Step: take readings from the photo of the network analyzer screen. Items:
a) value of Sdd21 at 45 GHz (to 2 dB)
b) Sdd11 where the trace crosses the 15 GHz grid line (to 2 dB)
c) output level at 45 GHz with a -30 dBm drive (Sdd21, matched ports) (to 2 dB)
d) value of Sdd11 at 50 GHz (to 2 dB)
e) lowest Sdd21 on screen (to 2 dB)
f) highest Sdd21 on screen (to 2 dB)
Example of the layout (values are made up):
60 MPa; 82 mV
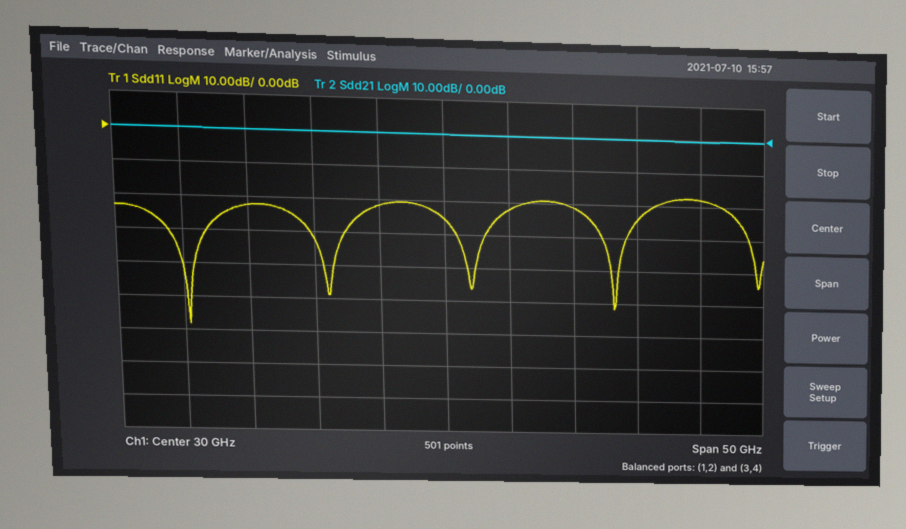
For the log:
0 dB; -22 dB; -30 dBm; -18 dB; 0 dB; 0 dB
